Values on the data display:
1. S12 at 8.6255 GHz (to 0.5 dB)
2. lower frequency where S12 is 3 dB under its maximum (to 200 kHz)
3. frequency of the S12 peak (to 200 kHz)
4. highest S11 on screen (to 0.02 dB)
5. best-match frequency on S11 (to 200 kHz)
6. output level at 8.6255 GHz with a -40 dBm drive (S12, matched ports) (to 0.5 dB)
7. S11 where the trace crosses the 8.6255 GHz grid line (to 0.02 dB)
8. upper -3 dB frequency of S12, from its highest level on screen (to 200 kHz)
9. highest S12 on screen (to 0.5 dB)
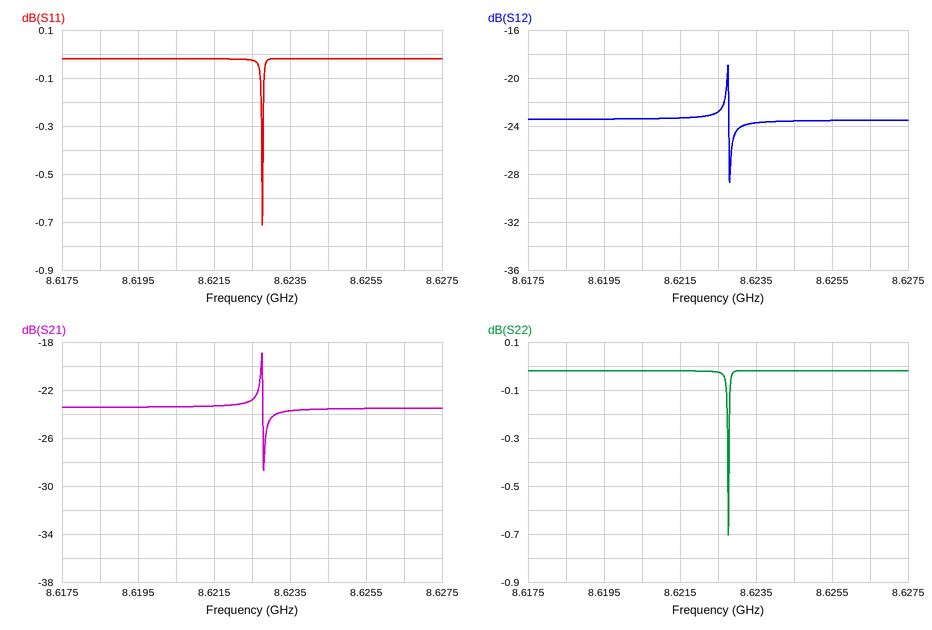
-23.5 dB
8.6226 GHz
8.6228 GHz
-0.02 dB
8.6228 GHz
-63.5 dBm
-0.02 dB
8.6228 GHz
-19.0 dB
